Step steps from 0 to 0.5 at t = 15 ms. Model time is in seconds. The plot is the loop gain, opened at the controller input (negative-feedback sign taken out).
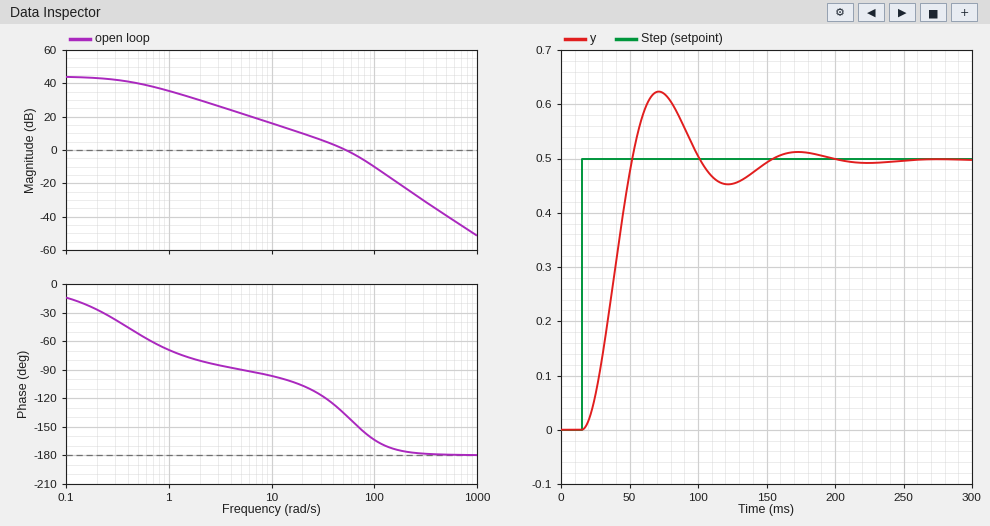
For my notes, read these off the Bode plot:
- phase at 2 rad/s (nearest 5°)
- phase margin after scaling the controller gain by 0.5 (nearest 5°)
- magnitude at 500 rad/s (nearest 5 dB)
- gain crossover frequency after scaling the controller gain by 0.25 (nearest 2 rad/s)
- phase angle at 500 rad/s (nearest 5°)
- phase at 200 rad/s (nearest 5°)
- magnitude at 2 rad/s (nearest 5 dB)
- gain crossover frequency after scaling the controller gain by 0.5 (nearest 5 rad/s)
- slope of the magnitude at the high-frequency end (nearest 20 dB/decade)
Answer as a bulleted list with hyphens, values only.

- -80°
- 65°
- -40 dB
- 16 rad/s
- -180°
- -175°
- 30 dB
- 30 rad/s
- -40 dB/decade
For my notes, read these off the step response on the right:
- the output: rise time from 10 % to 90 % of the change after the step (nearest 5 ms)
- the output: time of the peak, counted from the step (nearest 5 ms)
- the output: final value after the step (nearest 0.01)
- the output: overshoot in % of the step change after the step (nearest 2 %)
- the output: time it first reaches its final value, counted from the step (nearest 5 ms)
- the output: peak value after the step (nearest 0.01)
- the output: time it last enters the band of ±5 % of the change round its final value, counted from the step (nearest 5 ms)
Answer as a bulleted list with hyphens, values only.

- 25 ms
- 55 ms
- 0.50
- 26 %
- 35 ms
- 0.62
- 125 ms
